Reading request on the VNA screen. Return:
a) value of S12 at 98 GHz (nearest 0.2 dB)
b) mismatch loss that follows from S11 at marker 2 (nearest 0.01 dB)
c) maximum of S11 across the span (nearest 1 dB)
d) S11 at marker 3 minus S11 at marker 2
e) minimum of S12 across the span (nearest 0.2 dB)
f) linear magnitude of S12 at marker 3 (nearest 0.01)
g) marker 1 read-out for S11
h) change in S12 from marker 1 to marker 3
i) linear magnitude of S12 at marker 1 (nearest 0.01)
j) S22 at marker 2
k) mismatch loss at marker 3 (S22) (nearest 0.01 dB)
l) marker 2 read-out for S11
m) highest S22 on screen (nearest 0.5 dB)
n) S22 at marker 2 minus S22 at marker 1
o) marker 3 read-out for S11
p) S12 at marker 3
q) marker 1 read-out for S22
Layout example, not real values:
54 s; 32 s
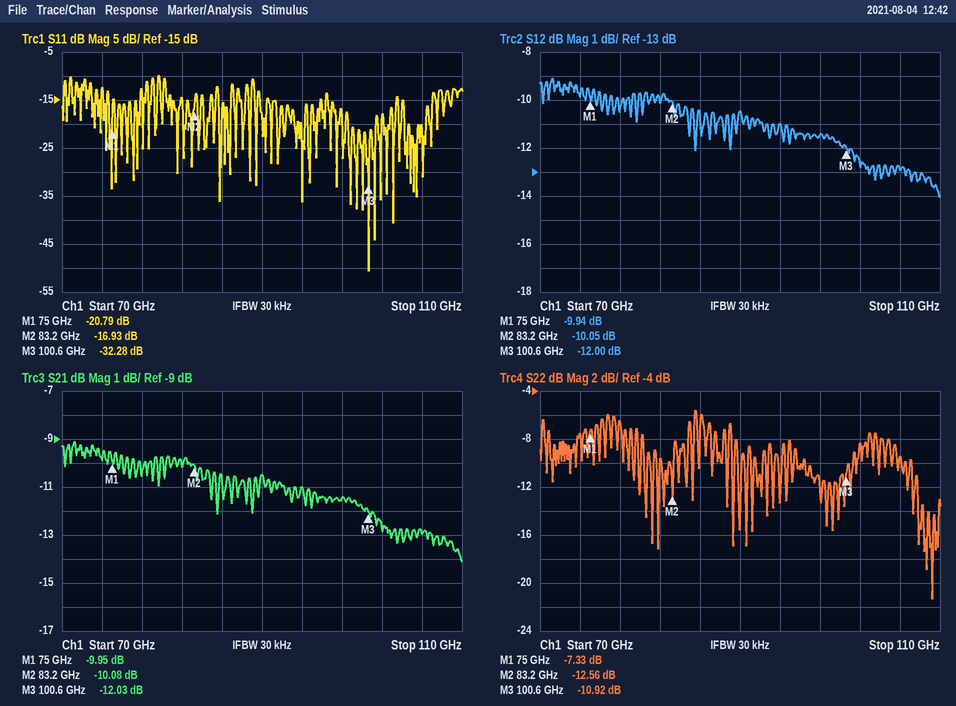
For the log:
-11.4 dB; 0.09 dB; -10 dB; -15.35 dB; -14.0 dB; 0.25; -20.79 dB; -2.06 dB; 0.32; -12.56 dB; 0.37 dB; -16.93 dB; -5.5 dB; -5.23 dB; -32.28 dB; -12.00 dB; -7.33 dB
